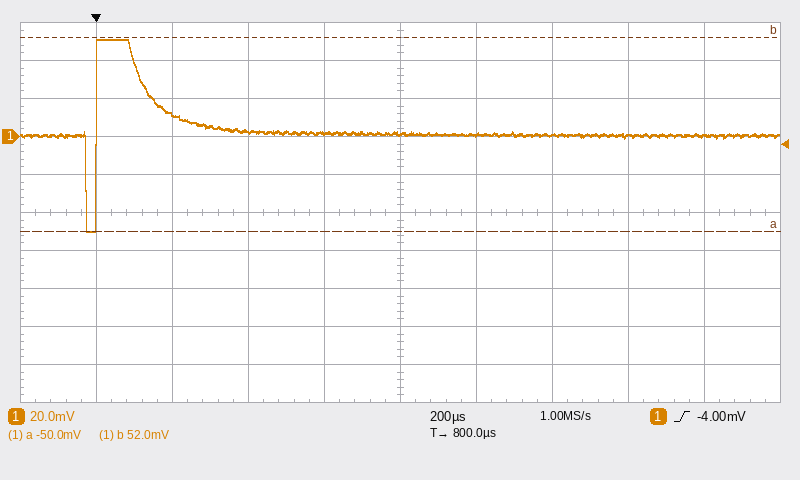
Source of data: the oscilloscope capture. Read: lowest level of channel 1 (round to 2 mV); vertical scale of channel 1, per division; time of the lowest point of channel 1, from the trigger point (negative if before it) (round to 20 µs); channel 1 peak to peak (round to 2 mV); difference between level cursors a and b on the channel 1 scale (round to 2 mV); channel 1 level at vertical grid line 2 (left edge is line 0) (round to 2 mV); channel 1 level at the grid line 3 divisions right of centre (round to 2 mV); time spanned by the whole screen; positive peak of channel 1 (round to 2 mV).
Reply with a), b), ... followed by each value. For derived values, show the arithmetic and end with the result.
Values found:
a) -50 mV
b) 20 mV
c) -20 µs
d) 52 mV − (-50 mV) = 102 mV
e) 102 mV
f) 12 mV
g) 0 mV
h) 2 ms
i) 52 mV
